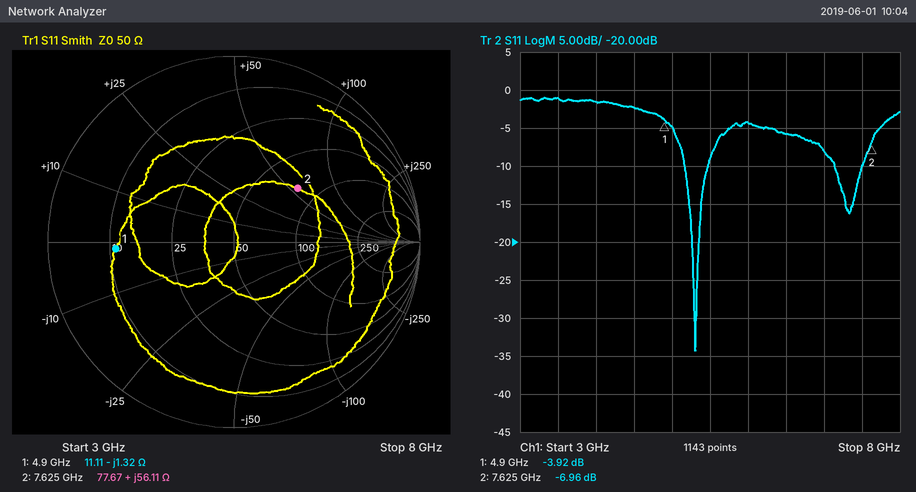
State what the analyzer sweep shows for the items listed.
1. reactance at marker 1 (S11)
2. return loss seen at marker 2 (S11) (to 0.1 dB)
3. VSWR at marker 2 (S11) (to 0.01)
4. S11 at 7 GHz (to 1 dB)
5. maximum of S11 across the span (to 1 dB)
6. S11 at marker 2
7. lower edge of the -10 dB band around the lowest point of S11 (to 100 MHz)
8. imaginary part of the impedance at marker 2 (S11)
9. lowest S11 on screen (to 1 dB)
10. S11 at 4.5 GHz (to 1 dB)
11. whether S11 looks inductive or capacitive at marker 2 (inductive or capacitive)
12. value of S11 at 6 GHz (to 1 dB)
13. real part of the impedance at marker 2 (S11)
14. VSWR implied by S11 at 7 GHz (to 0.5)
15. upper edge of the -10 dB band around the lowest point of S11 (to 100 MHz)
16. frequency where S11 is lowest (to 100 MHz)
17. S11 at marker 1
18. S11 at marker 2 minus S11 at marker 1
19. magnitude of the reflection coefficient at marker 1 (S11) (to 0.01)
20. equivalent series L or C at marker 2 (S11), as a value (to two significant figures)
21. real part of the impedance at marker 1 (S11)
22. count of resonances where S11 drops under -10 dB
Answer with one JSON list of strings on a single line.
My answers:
["-1.32 Ω", "7.0 dB", "2.63", "-8 dB", "-1 dB", "-6.96 dB", "5.2 GHz", "+56.11 Ω", "-34 dB", "-2 dB", "inductive", "-4 dB", "77.67 Ω", "2.5", "5.5 GHz", "5.3 GHz", "-3.92 dB", "-3.04 dB", "0.64", "1.2 nH", "11.11 Ω", "2"]
